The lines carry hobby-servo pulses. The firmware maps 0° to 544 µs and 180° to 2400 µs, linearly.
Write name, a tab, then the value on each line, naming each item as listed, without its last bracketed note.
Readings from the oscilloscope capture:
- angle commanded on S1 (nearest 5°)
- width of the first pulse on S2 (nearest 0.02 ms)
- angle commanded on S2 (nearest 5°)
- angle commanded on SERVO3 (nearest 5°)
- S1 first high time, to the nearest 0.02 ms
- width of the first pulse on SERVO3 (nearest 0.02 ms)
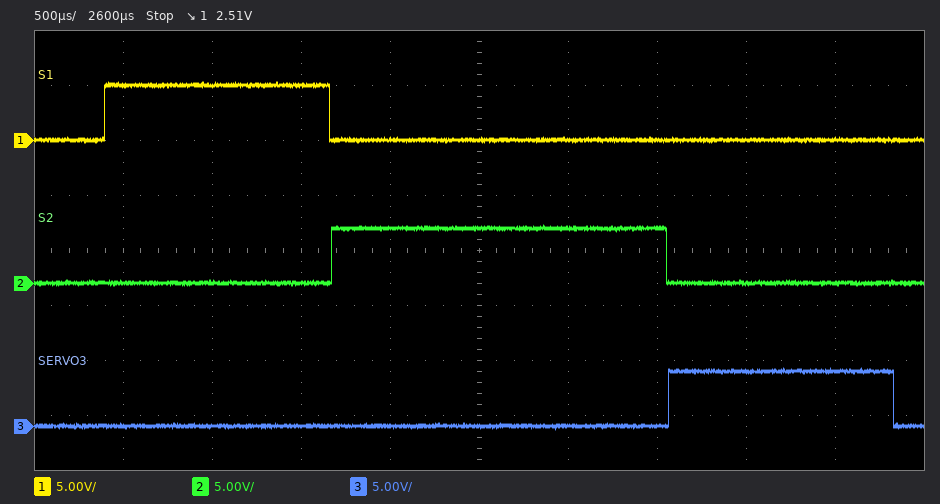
angle commanded on S1	70°
width of the first pulse on S2	1.88 ms
angle commanded on S2	130°
angle commanded on SERVO3	70°
S1 first high time, to the nearest 0.02 ms	1.26 ms
width of the first pulse on SERVO3	1.26 ms
